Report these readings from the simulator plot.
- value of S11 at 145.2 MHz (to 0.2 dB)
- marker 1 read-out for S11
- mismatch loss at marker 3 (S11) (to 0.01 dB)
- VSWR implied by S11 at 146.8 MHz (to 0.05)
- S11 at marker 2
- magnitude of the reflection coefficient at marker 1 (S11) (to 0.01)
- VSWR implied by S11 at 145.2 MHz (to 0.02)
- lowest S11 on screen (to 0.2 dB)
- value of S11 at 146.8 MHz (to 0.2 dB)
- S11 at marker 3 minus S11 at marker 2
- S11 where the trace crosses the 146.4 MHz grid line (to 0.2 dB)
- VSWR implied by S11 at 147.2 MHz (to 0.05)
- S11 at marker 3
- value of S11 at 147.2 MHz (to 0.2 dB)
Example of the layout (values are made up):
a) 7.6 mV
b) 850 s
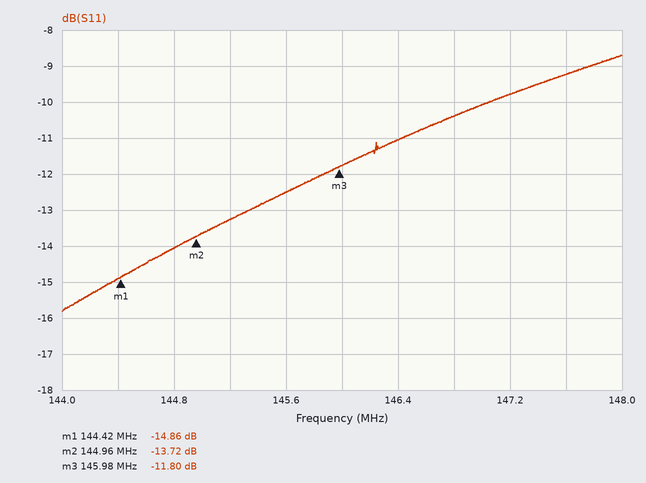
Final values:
a) -13.2 dB
b) -14.86 dB
c) 0.30 dB
d) 1.85
e) -13.72 dB
f) 0.18
g) 1.56
h) -15.8 dB
i) -10.4 dB
j) 1.92 dB
k) -11.0 dB
l) 1.95
m) -11.80 dB
n) -9.8 dB
